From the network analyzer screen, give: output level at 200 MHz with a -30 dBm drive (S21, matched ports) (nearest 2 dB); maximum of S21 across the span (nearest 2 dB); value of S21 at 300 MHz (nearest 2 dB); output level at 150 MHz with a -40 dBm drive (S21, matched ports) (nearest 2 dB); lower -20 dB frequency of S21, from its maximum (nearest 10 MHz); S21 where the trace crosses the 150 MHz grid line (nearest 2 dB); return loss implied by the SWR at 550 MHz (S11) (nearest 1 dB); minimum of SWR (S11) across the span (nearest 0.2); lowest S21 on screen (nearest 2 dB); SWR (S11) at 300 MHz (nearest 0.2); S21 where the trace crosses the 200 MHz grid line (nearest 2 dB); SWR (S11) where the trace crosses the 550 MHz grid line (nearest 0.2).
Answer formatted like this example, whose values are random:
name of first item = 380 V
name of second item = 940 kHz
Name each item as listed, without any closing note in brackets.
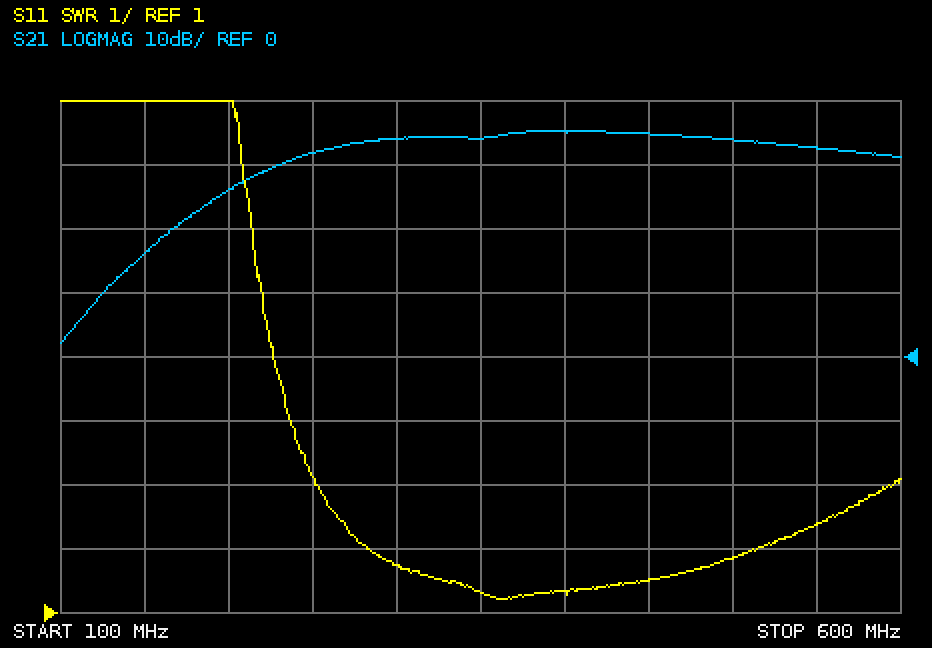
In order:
output level at 200 MHz with a -30 dBm drive (S21, matched ports) = -4 dBm
maximum of S21 across the span = 36 dB
value of S21 at 300 MHz = 34 dB
output level at 150 MHz with a -40 dBm drive (S21, matched ports) = -24 dBm
lower -20 dB frequency of S21, from its maximum = 150 MHz
S21 where the trace crosses the 150 MHz grid line = 16 dB
return loss implied by the SWR at 550 MHz (S11) = 8 dB
minimum of SWR (S11) across the span = 1.2
lowest S21 on screen = 2 dB
SWR (S11) at 300 MHz = 1.8
S21 where the trace crosses the 200 MHz grid line = 26 dB
SWR (S11) where the trace crosses the 550 MHz grid line = 2.4
